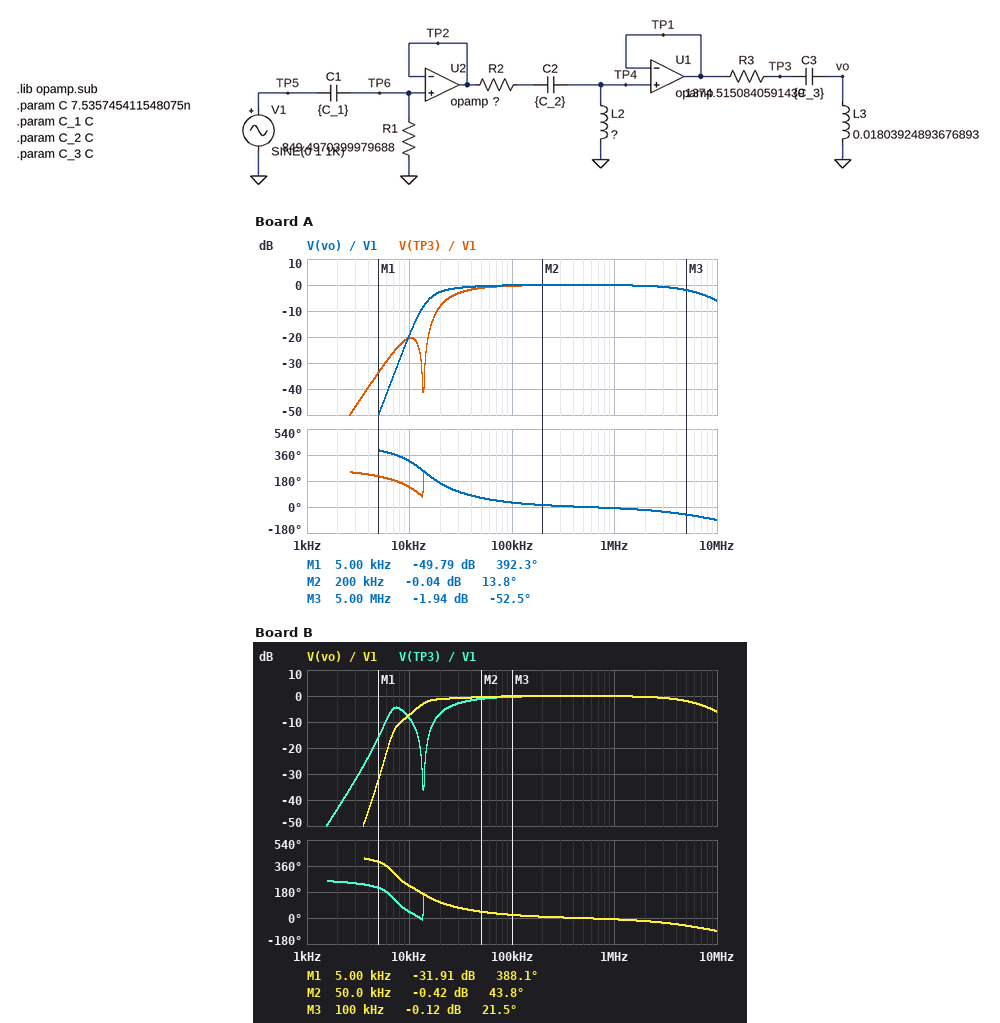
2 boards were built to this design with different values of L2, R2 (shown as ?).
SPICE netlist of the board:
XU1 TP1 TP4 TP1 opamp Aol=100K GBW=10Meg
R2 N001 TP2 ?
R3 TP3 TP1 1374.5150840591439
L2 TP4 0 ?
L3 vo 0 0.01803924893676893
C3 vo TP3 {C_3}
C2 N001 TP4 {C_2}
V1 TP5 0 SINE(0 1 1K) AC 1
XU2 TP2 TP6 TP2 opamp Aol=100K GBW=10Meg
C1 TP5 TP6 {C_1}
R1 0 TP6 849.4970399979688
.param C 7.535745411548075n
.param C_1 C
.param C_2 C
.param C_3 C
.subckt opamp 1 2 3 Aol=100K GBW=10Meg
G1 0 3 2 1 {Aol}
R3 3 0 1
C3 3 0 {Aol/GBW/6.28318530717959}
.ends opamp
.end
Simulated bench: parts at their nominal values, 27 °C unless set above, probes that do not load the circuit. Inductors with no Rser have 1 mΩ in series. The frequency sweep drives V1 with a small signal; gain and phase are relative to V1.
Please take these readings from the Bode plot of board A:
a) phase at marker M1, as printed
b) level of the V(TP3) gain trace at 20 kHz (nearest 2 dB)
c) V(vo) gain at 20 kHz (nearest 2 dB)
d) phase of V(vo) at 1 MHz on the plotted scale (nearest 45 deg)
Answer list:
392.3 deg
-8 dB
-2 dB
0 deg
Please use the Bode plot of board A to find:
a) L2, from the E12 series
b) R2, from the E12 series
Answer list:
15 mH
1.8 kΩ
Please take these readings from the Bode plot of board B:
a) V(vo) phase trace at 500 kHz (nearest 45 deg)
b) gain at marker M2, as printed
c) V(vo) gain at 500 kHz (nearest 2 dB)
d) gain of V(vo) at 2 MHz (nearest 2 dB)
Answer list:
0 deg
-0.42 dB
0 dB
0 dB
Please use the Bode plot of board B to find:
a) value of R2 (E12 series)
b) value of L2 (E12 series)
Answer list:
1.2 kΩ
68 mH
